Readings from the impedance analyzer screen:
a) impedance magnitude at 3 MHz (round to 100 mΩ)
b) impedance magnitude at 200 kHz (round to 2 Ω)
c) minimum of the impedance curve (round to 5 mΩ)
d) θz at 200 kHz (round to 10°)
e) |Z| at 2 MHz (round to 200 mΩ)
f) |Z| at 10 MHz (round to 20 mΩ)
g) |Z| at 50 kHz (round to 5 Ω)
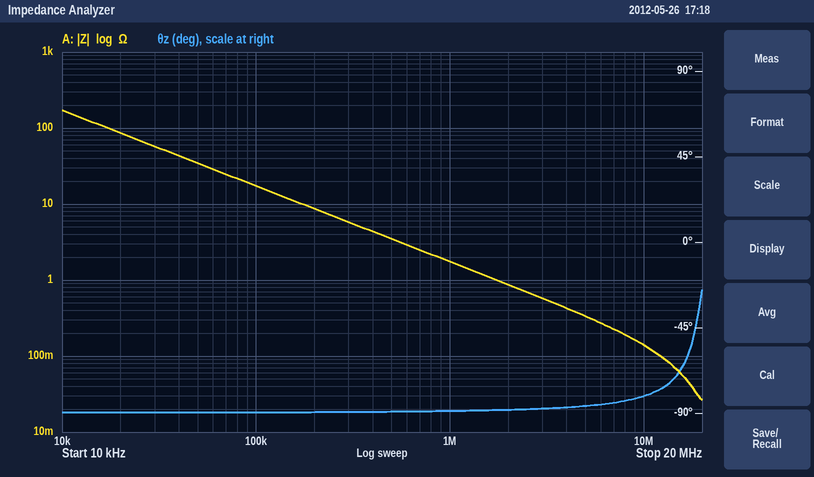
600 mΩ
8 Ω
25 mΩ
-90°
800 mΩ
140 mΩ
35 Ω
